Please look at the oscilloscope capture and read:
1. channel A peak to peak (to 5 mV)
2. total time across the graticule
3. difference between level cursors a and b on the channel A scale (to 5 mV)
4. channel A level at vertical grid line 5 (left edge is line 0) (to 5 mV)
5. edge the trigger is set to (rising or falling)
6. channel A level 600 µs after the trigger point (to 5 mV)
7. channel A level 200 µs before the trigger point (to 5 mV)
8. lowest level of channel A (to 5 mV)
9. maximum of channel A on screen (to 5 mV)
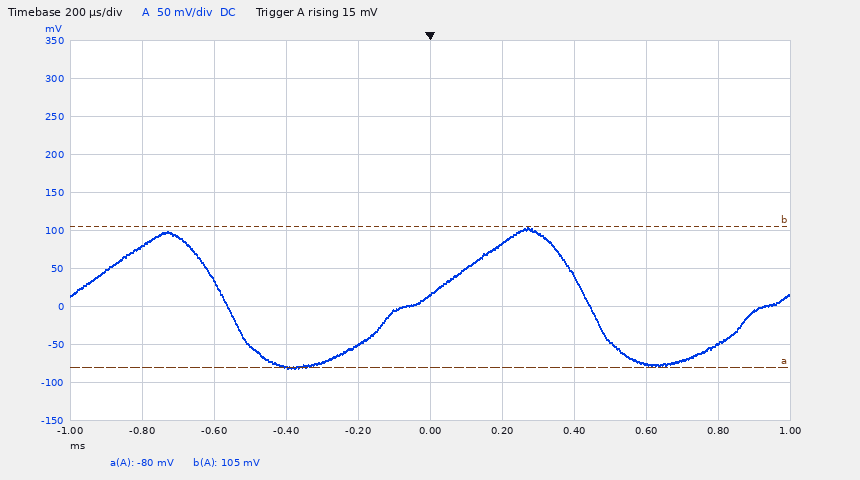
185 mV
2 ms
185 mV
15 mV
rising
-75 mV
-50 mV
-80 mV
105 mV
